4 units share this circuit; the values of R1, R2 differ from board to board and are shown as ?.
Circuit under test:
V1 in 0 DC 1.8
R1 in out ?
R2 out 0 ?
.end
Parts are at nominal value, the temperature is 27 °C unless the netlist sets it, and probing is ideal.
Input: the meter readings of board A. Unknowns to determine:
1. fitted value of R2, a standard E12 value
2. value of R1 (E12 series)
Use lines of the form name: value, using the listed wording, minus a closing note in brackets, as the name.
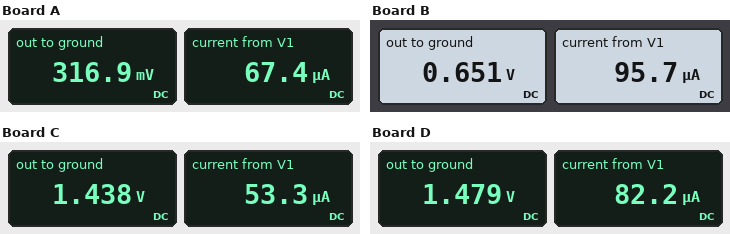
fitted value of R2, a standard E12 value: 4.7 kΩ
value of R1: 22 kΩ
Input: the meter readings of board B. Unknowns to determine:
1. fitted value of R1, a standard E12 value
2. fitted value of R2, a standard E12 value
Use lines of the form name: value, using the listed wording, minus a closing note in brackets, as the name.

fitted value of R1, a standard E12 value: 12 kΩ
fitted value of R2, a standard E12 value: 6.8 kΩ
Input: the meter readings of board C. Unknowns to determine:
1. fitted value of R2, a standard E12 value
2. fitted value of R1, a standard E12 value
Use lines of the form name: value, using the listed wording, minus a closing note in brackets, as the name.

fitted value of R2, a standard E12 value: 27 kΩ
fitted value of R1, a standard E12 value: 6.8 kΩ
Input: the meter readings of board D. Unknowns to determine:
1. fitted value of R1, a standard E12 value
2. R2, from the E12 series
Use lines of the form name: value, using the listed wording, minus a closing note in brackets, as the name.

fitted value of R1, a standard E12 value: 3.9 kΩ
R2, from the E12 series: 18 kΩ
